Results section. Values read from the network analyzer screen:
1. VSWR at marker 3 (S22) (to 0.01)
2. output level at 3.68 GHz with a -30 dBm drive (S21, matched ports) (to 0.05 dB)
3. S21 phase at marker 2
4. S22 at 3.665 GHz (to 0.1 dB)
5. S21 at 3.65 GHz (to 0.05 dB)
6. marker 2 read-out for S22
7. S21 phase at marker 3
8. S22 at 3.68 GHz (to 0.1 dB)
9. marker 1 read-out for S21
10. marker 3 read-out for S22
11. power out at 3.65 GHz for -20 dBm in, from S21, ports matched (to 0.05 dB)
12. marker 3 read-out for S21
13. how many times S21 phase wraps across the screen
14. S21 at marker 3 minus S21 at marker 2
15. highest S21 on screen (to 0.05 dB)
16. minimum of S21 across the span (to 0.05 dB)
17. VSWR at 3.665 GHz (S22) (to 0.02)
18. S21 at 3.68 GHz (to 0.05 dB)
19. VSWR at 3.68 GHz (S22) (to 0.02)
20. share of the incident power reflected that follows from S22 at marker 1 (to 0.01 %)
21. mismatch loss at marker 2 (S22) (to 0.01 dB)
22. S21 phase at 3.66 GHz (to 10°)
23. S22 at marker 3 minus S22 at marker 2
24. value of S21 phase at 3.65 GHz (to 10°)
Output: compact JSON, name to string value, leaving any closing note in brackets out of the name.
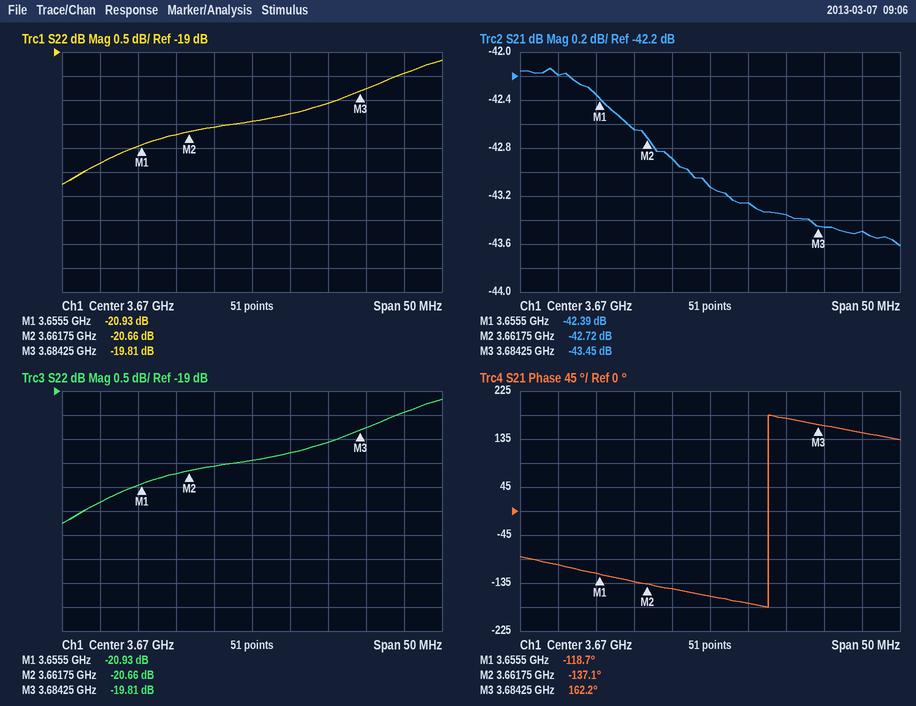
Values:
{"VSWR at marker 3 (S22)": "1.23", "output level at 3.68 GHz with a -30 dBm drive (S21, matched ports)": "-73.35 dBm", "S21 phase at marker 2": "-137.1°", "S22 at 3.665 GHz": "-20.6 dB", "S21 at 3.65 GHz": "-42.20 dB", "marker 2 read-out for S22": "-20.66 dB", "S21 phase at marker 3": "162.2°", "S22 at 3.68 GHz": "-20.1 dB", "marker 1 read-out for S21": "-42.39 dB", "marker 3 read-out for S22": "-19.81 dB", "power out at 3.65 GHz for -20 dBm in, from S21, ports matched": "-62.20 dBm", "marker 3 read-out for S21": "-43.45 dB", "how many times S21 phase wraps across the screen": "1", "S21 at marker 3 minus S21 at marker 2": "-0.73 dB", "highest S21 on screen": "-42.15 dB", "minimum of S21 across the span": "-43.60 dB", "VSWR at 3.665 GHz (S22)": "1.20", "S21 at 3.68 GHz": "-43.35 dB", "VSWR at 3.68 GHz (S22)": "1.22", "share of the incident power reflected that follows from S22 at marker 1": "0.81 %", "mismatch loss at marker 2 (S22)": "0.04 dB", "S21 phase at 3.66 GHz": "-130°", "S22 at marker 3 minus S22 at marker 2": "0.85 dB", "value of S21 phase at 3.65 GHz": "-100°"}
